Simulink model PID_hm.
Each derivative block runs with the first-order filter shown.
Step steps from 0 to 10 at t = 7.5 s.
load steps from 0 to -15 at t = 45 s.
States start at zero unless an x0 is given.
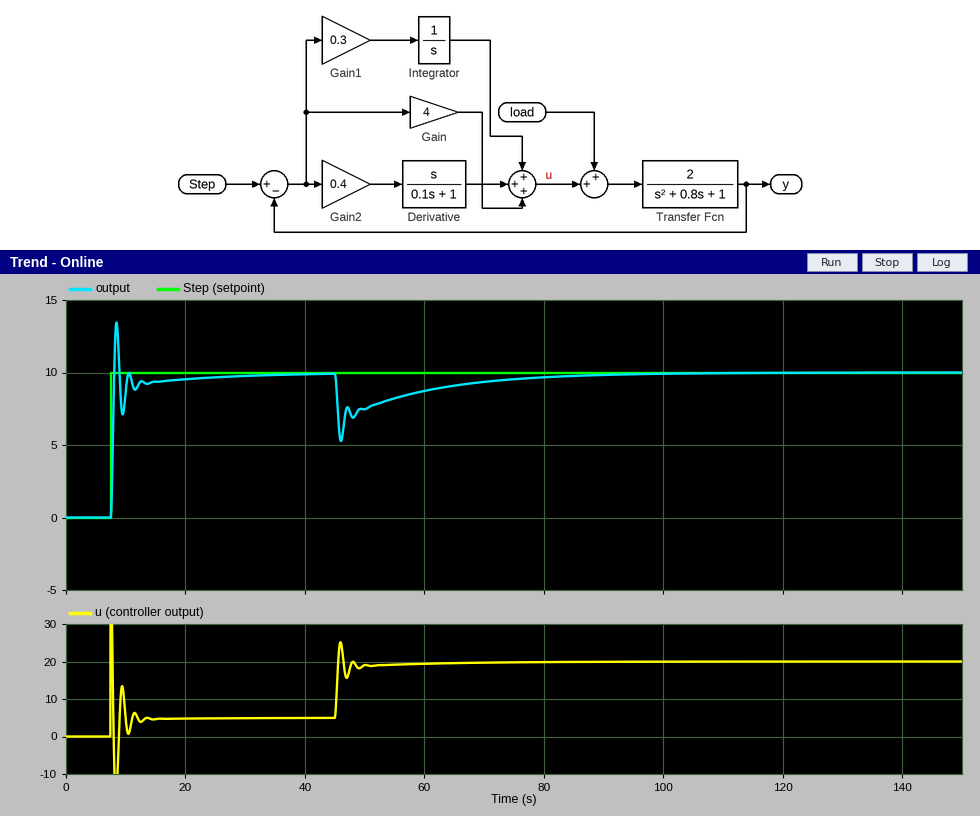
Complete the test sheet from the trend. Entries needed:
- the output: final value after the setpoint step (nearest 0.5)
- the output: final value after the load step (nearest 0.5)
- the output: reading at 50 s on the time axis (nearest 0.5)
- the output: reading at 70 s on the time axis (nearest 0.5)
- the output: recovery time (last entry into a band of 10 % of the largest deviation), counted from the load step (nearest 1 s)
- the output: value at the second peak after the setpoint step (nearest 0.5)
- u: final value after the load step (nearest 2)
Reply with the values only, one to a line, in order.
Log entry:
10.0
10.0
7.5
9.5
30 s
10.0
20
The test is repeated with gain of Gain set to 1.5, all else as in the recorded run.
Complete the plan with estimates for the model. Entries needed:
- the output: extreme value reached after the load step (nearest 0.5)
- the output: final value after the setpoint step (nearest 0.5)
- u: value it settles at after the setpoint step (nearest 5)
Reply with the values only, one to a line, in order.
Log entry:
1.0
10.0
5
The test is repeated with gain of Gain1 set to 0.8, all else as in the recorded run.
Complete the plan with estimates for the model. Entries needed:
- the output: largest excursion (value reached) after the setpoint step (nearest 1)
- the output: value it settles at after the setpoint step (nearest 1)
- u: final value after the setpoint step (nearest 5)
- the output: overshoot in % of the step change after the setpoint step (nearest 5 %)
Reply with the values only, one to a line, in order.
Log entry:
14
10
5
40 %
